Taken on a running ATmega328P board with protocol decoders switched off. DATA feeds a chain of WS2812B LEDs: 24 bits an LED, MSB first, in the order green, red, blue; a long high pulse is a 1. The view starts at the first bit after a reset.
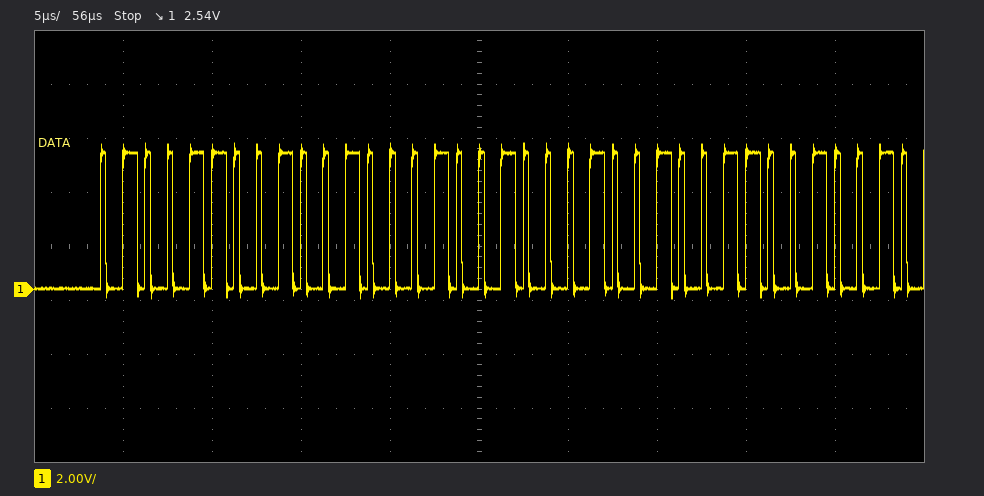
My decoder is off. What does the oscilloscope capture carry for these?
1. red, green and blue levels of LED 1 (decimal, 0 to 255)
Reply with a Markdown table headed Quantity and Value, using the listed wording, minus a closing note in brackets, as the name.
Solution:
| Quantity | Value |
|---|---|
| red, green and blue levels of LED 1 | 145, 76, 34 |
